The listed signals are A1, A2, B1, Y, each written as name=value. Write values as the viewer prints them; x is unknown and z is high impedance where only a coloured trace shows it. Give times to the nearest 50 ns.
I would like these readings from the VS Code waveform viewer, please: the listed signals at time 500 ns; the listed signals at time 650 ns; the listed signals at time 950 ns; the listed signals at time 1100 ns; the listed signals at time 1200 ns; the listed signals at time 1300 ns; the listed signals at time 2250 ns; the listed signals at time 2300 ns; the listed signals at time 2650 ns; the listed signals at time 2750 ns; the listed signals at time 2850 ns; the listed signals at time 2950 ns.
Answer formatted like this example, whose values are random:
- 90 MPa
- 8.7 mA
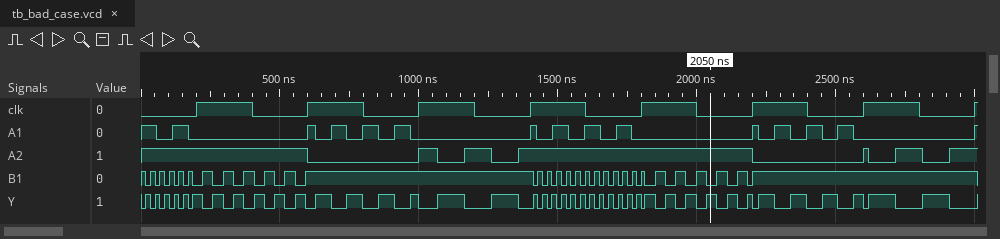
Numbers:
- A1=0, A2=1, B1=0, Y=1
- A1=0, A2=0, B1=1, Y=1
- A1=1, A2=0, B1=1, Y=0
- A1=0, A2=0, B1=1, Y=1
- A1=0, A2=1, B1=1, Y=0
- A1=0, A2=0, B1=1, Y=1
- A1=0, A2=0, B1=1, Y=1
- A1=1, A2=0, B1=1, Y=0
- A1=0, A2=0, B1=1, Y=1
- A1=0, A2=1, B1=1, Y=0
- A1=0, A2=0, B1=1, Y=1
- A1=0, A2=1, B1=1, Y=0
